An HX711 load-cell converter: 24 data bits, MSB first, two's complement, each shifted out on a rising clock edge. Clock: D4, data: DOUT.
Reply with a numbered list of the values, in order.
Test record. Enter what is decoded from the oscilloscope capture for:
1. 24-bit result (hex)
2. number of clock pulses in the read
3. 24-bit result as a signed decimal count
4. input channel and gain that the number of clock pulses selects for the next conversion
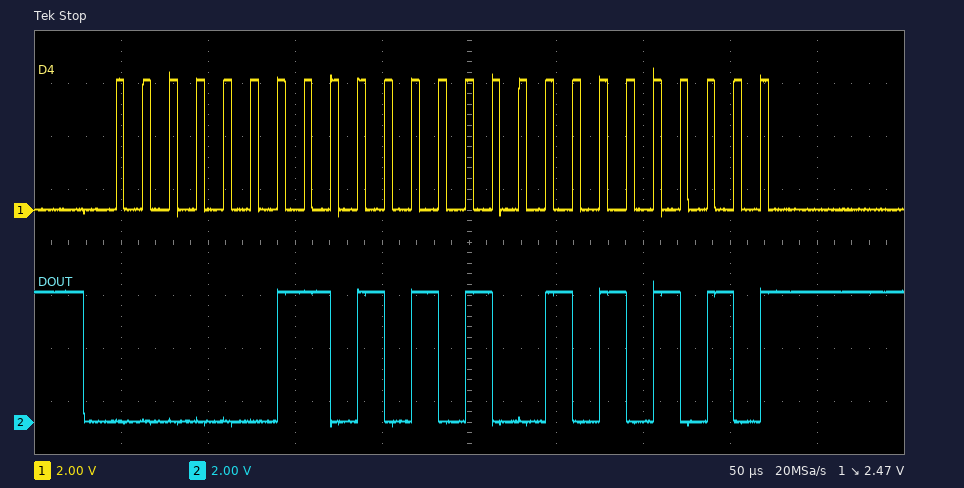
1. 0x0354AA
2. 25
3. 218282
4. channel A, gain 128
